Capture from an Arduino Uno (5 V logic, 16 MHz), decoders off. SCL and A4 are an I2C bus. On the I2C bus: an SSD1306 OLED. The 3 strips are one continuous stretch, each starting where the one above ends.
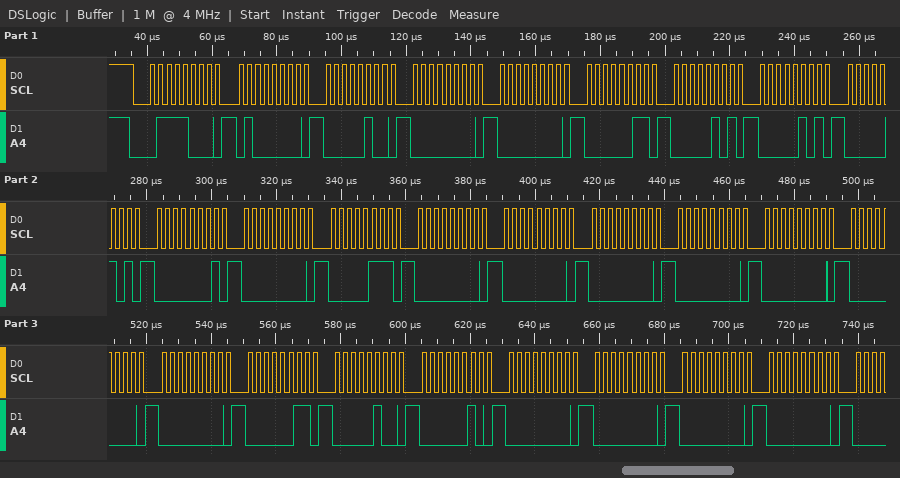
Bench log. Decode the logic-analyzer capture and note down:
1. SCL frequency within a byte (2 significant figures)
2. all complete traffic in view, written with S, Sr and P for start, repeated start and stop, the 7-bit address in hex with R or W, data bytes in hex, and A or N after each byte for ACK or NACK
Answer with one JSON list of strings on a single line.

["400 kHz", "S 3CW A 40 A 04 A 00 A 00 A 03 A 05 A 05 A 05 A 01 A 00 A 07 A 00 A 00 A 00 A 00 A 00 A 00 A 00 A 03 A 04 A 02 A 00 A 00 A 00 A 00 A"]
